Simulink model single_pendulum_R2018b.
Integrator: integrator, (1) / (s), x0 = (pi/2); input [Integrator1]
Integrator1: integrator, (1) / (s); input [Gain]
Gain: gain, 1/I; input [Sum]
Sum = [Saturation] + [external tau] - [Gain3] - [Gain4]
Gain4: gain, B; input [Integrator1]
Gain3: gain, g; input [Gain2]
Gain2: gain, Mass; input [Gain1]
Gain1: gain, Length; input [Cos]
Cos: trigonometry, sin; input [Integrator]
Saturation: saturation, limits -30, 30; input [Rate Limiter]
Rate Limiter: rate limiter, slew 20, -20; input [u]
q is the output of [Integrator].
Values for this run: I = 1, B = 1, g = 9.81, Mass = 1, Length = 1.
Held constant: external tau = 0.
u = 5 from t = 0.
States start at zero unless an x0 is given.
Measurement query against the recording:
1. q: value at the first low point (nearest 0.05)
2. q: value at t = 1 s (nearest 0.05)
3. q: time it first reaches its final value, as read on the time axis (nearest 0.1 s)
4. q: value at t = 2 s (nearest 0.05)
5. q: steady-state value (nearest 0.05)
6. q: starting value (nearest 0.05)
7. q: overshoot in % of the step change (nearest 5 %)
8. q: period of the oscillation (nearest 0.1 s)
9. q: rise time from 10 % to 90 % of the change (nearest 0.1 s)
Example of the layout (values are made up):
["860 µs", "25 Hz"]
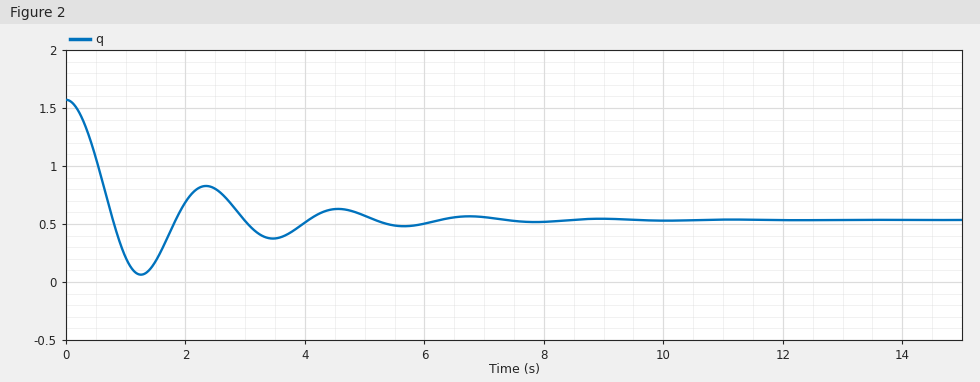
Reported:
["0.05", "0.20", "0.8 s", "0.70", "0.55", "1.55", "45 %", "2.2 s", "0.5 s"]
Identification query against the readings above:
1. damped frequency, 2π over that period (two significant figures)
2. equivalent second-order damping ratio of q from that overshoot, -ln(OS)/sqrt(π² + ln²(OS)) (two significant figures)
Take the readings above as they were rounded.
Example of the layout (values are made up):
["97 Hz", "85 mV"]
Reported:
["2.9 rad/s", "0.25"]
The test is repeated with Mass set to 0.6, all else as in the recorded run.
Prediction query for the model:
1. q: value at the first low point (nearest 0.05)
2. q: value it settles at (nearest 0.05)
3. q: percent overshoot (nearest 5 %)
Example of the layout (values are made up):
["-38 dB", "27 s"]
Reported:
["0.85", "1.00", "30 %"]
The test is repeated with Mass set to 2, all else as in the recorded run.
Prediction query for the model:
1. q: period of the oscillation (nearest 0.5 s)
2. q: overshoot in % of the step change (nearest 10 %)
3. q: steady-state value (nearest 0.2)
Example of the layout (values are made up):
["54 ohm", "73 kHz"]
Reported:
["1.5 s", "60 %", "0.2"]
